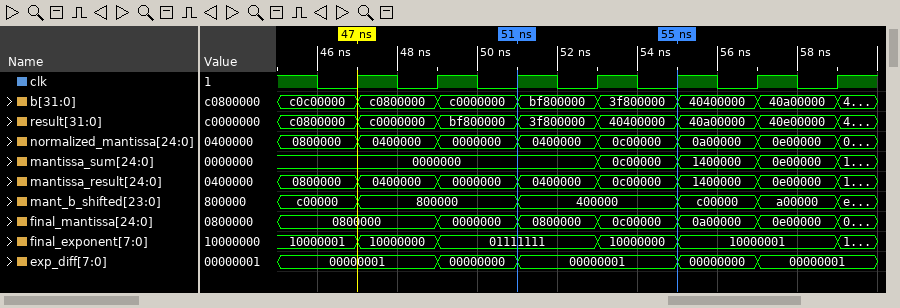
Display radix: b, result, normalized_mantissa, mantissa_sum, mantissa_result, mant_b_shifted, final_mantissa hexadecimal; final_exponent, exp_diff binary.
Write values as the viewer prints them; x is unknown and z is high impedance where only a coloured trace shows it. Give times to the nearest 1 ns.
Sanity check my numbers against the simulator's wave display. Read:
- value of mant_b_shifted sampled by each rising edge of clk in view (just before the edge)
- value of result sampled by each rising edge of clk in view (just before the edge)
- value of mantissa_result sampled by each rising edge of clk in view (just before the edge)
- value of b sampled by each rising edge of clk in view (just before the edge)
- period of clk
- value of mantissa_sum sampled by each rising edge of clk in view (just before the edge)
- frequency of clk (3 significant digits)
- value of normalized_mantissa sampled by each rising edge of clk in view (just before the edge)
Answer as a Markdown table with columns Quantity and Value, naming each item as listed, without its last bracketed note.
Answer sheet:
| Quantity | Value |
|---|---|
| value of mant_b_shifted sampled by each rising edge of clk in view | c00000, 800000, 800000, 400000, 400000, c00000, a00000 |
| value of result sampled by each rising edge of clk in view | c0800000, c0000000, bf800000, 3f800000, 40400000, 40a00000, 40e00000 |
| value of mantissa_result sampled by each rising edge of clk in view | 0800000, 0400000, 0000000, 0400000, 0c00000, 1400000, 0e00000 |
| value of b sampled by each rising edge of clk in view | c0c00000, c0800000, c0000000, bf800000, 3f800000, 40400000, 40a00000 |
| period of clk | 2 ns |
| value of mantissa_sum sampled by each rising edge of clk in view | 0000000, 0000000, 0000000, 0000000, 0c00000, 1400000, 0e00000 |
| frequency of clk | 500 MHz |
| value of normalized_mantissa sampled by each rising edge of clk in view | 0800000, 0400000, 0000000, 0400000, 0c00000, 0a00000, 0e00000 |
